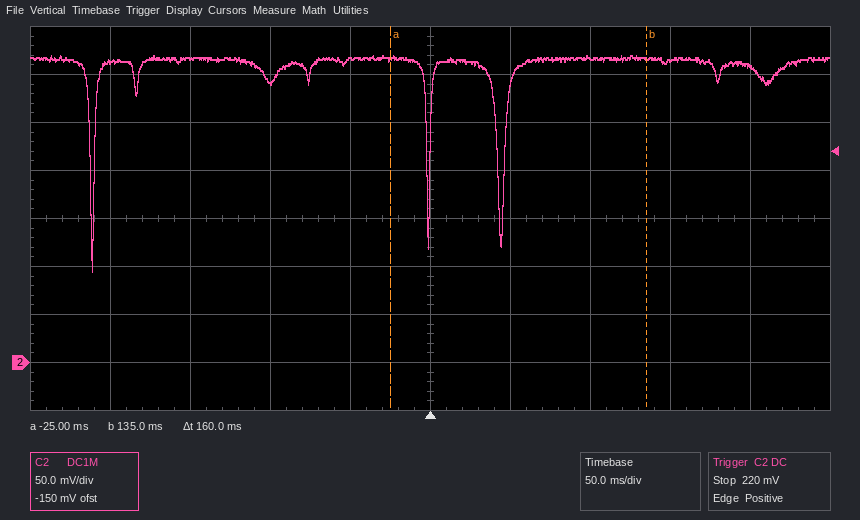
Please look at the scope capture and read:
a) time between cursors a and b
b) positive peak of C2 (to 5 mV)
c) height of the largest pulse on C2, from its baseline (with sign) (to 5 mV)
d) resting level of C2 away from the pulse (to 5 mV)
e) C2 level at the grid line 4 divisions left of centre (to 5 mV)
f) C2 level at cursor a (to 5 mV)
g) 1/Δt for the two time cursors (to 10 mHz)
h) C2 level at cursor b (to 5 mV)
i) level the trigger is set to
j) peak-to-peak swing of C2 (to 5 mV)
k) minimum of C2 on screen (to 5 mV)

160 ms
320 mV
-220 mV
315 mV
315 mV
315 mV
6.25 Hz
315 mV
220 mV
225 mV
95 mV
